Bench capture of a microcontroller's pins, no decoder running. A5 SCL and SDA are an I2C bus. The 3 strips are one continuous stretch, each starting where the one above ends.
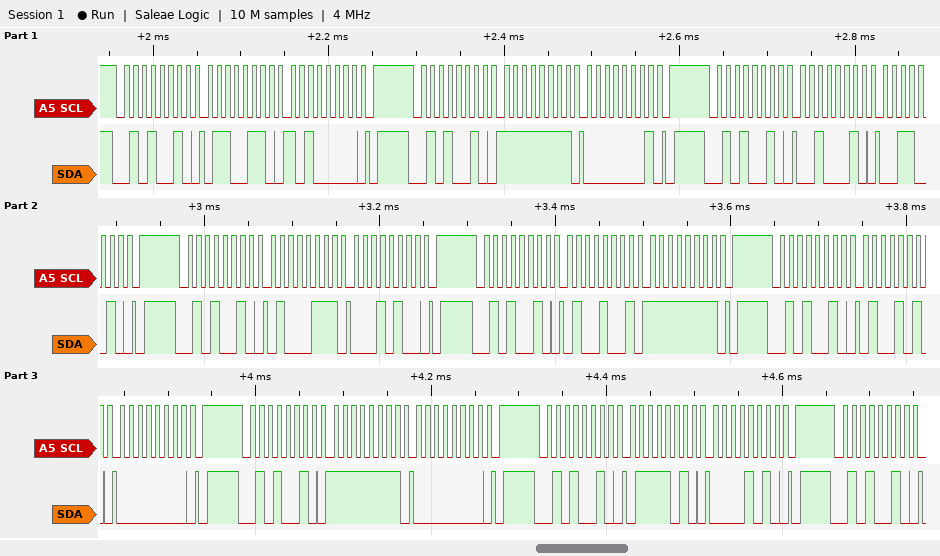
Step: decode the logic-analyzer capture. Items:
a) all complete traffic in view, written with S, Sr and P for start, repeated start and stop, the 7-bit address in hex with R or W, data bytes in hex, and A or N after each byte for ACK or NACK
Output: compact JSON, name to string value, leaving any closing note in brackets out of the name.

{"all complete traffic in view, written with S, Sr and P for start, repeated start and stop, the 7-bit address in hex with R or W, data bytes in hex, and A or N after each byte for ACK or NACK": "S 29W A 66 A A0 A P S 29W A FF A 01 A P S 29W A 22 A 32 A P S 29W A 47 A 14 A P S 29W A 49 A FF A P S 29W A 4A A 00 A P S 29W A FF A 00 A P S 29W A 7A A 0A A P S 29W A"}
